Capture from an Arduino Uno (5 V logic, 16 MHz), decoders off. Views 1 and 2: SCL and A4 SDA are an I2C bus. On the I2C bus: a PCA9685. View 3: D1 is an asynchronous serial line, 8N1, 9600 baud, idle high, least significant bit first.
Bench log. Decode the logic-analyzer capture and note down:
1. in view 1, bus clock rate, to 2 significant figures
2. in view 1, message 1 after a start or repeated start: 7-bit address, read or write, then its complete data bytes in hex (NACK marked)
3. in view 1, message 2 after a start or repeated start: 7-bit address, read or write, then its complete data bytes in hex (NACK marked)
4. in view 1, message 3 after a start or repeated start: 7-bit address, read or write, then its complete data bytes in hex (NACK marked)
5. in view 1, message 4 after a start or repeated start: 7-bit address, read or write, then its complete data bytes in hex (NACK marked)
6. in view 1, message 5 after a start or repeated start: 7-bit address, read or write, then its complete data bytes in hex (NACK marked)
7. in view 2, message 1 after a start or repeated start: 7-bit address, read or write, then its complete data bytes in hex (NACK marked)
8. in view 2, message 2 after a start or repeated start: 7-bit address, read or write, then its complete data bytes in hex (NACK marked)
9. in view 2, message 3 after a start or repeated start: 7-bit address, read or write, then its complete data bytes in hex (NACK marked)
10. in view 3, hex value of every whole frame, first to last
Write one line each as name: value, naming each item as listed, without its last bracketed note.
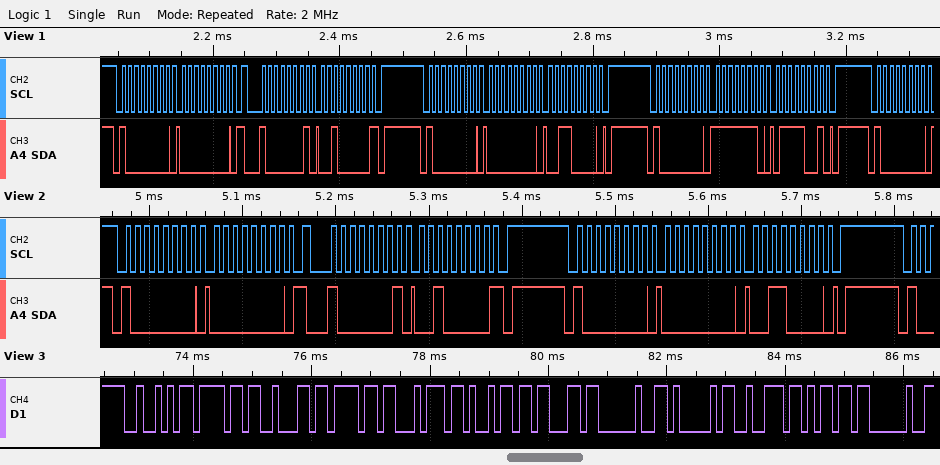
in view 1, bus clock rate, to 2 significant figures: 100 kHz
in view 1, message 1 after a start or repeated start: 7-bit address, read or write, then its complete data bytes in hex: 0x40 write: 00
in view 1, message 2 after a start or repeated start: 7-bit address, read or write, then its complete data bytes in hex: 0x40 read: 20 NACK
in view 1, message 3 after a start or repeated start: 7-bit address, read or write, then its complete data bytes in hex: 0x40 write: 00 30
in view 1, message 4 after a start or repeated start: 7-bit address, read or write, then its complete data bytes in hex: 0x40 write: FE 79
in view 1, message 5 after a start or repeated start: 7-bit address, read or write, then its complete data bytes in hex: 0x40 write
in view 2, message 1 after a start or repeated start: 7-bit address, read or write, then its complete data bytes in hex: 0x40 write: 00
in view 2, message 2 after a start or repeated start: 7-bit address, read or write, then its complete data bytes in hex: 0x40 read: 20 NACK
in view 2, message 3 after a start or repeated start: 7-bit address, read or write, then its complete data bytes in hex: 0x40 write: 00 30
in view 3, hex value of every whole frame, first to last: 0x52 0x6F 0x62 0x6F 0x74 0x69 0x63 0x20 0x41 0x72 0x6D 0x20
